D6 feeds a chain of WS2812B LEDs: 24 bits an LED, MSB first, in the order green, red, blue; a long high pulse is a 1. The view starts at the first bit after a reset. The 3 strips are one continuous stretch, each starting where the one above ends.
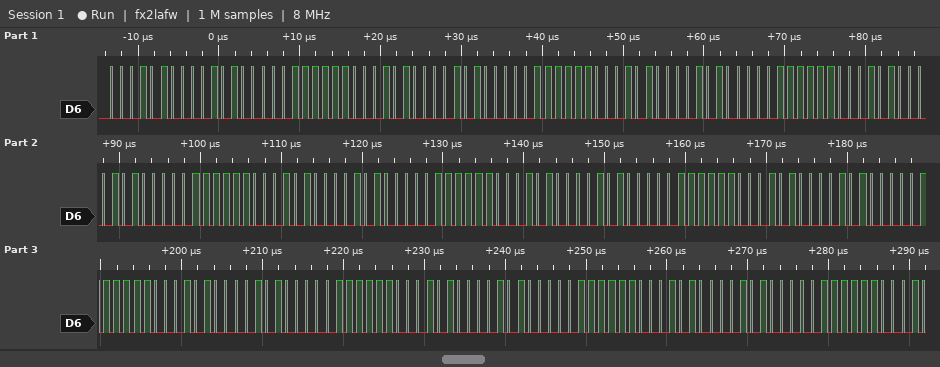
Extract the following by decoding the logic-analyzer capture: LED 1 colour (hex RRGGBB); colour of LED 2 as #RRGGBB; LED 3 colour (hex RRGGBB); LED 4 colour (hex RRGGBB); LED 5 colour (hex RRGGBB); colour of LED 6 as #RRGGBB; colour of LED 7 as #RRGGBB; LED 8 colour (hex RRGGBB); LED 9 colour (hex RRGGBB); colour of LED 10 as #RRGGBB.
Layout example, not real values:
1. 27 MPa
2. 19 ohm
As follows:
1. #28143F
2. #28143F
3. #28143F
4. #28143F
5. #28143F
6. #28143F
7. #28143F
8. #28143F
9. #28143F
10. #28143F
